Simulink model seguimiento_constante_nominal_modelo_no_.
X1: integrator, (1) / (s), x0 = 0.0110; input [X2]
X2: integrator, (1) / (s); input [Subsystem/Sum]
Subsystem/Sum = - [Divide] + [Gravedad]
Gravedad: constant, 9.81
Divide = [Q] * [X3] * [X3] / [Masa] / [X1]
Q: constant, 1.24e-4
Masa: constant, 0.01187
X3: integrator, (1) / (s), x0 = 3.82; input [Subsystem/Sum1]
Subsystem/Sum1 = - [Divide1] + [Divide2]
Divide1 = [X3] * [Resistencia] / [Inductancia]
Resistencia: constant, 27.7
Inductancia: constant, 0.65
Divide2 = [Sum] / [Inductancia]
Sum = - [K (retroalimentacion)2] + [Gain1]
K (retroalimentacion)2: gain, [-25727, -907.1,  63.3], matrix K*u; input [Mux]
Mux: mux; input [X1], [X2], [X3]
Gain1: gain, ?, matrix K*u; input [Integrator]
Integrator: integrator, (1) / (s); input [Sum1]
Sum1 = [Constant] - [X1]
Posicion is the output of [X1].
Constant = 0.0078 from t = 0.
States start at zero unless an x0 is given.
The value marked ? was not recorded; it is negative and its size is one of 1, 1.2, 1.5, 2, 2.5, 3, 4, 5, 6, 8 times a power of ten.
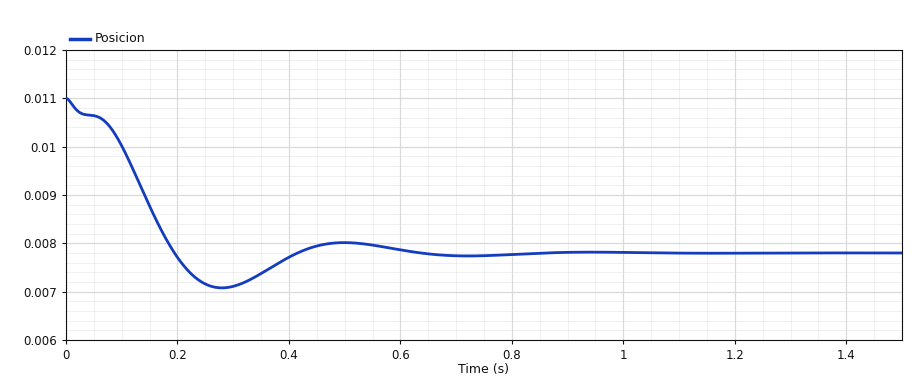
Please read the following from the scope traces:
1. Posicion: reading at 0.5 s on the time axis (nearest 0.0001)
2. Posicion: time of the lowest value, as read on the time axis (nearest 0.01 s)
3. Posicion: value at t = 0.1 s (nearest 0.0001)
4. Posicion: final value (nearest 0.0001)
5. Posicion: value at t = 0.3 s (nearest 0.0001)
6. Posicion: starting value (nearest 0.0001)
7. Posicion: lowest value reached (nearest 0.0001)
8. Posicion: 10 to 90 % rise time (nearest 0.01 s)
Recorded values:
0.0080
0.28 s
0.0100
0.0078
0.0071
0.0110
0.0071
0.15 s
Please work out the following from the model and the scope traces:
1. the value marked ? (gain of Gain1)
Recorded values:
-150000
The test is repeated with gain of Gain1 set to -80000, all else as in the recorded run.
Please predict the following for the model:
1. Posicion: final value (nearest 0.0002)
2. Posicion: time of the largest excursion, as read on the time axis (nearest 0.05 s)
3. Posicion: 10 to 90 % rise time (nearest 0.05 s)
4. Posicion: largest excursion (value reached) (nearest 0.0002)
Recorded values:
0.0078
0.45 s
0.20 s
0.0076
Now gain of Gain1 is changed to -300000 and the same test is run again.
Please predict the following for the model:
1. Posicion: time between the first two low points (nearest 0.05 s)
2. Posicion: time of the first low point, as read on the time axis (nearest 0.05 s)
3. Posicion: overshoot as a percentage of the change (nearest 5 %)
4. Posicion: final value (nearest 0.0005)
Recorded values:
0.30 s
0.20 s
50 %
0.0080
